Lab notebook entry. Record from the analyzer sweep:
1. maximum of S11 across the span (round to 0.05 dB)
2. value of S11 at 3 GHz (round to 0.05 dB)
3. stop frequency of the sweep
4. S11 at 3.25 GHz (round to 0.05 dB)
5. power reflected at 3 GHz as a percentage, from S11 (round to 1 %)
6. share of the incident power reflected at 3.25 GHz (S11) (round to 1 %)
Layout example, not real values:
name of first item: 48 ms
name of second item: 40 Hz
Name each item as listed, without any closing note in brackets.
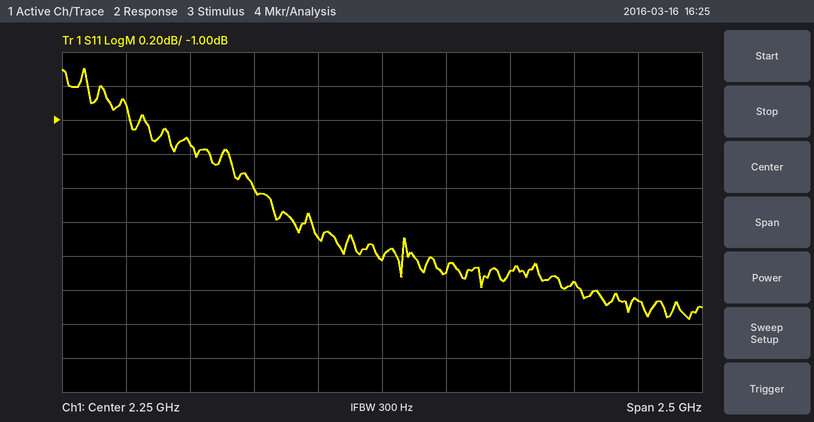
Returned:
maximum of S11 across the span: -0.70 dB
value of S11 at 3 GHz: -1.95 dB
stop frequency of the sweep: 3.5 GHz
S11 at 3.25 GHz: -2.05 dB
power reflected at 3 GHz as a percentage, from S11: 64 %
share of the incident power reflected at 3.25 GHz (S11): 62 %
